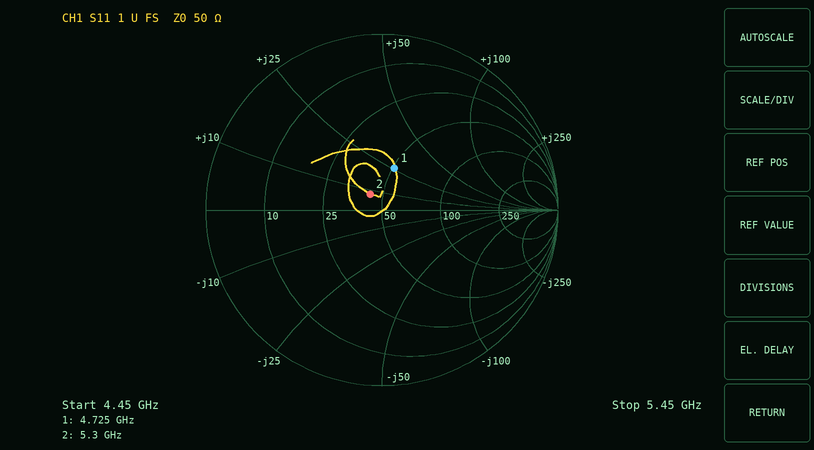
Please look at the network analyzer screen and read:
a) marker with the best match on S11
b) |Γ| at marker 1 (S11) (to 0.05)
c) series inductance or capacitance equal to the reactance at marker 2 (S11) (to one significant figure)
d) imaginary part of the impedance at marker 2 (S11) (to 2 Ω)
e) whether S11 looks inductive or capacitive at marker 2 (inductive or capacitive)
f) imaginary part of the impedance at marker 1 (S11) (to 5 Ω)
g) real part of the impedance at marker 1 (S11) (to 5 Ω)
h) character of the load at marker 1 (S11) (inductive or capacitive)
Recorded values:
marker 2
0.25
200 pH
+8 Ω
inductive
+25 Ω
50 Ω
inductive
